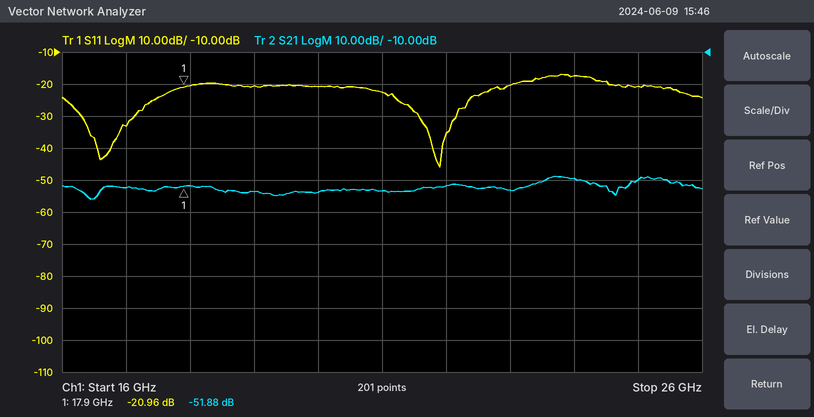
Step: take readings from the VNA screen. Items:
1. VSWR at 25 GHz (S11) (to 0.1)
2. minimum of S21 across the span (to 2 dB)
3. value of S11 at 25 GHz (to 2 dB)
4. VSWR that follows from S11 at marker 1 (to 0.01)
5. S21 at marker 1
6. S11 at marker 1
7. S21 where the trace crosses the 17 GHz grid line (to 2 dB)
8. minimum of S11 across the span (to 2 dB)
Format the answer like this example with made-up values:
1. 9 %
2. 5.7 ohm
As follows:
1. 1.2
2. -56 dB
3. -20 dB
4. 1.20
5. -51.88 dB
6. -20.96 dB
7. -52 dB
8. -46 dB
